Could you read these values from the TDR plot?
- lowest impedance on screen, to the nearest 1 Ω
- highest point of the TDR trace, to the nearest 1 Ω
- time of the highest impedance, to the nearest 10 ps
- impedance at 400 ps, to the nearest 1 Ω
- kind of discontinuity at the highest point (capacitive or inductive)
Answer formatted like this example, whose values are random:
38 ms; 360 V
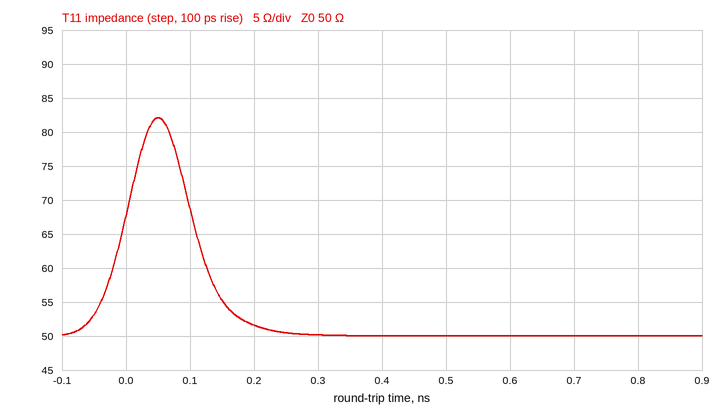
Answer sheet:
50 Ω; 82 Ω; 50 ps; 50 Ω; inductive
